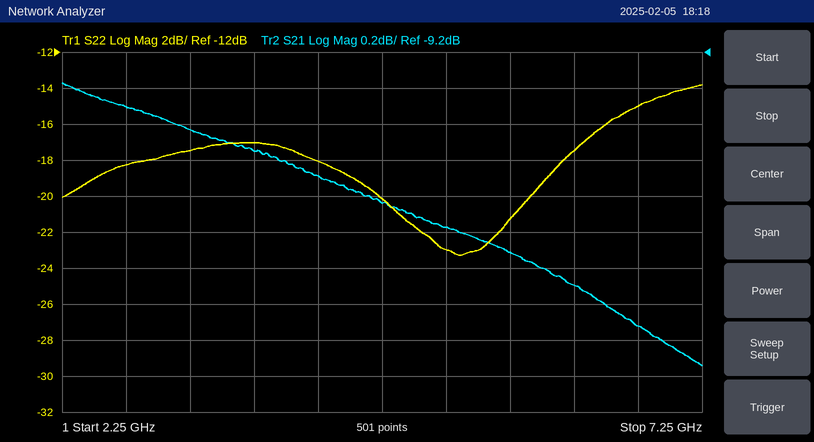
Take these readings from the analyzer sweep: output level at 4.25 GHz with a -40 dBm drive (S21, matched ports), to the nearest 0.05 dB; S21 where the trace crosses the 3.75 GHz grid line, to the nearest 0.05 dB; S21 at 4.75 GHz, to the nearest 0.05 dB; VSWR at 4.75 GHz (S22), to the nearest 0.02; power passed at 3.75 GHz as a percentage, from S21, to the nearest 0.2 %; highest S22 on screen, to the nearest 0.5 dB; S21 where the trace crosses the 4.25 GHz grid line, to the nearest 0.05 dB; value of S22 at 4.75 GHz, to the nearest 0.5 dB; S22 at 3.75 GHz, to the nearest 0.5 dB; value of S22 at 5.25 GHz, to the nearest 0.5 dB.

-49.90 dBm
-9.75 dB
-10.05 dB
1.22
10.6 %
-14.0 dB
-9.90 dB
-20.0 dB
-17.0 dB
-23.0 dB
